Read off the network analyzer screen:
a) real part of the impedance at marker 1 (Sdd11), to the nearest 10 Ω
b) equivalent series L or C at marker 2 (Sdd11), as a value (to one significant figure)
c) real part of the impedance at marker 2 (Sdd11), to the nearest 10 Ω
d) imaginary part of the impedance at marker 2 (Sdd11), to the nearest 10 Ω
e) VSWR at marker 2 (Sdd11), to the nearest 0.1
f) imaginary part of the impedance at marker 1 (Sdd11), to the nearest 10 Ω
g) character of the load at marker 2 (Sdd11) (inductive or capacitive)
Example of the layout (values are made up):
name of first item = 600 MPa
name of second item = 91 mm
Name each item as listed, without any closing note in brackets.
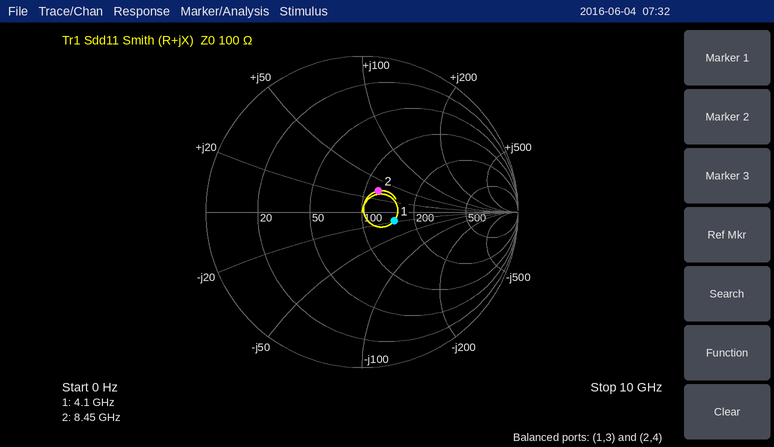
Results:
real part of the impedance at marker 1 (Sdd11), to the nearest 10 Ω = 150 Ω
equivalent series L or C at marker 2 (Sdd11), as a value = 600 pH
real part of the impedance at marker 2 (Sdd11), to the nearest 10 Ω = 120 Ω
imaginary part of the impedance at marker 2 (Sdd11), to the nearest 10 Ω = +30 Ω
VSWR at marker 2 (Sdd11), to the nearest 0.1 = 1.4
imaginary part of the impedance at marker 1 (Sdd11), to the nearest 10 Ω = -20 Ω
character of the load at marker 2 (Sdd11) = inductive
